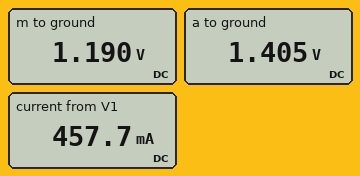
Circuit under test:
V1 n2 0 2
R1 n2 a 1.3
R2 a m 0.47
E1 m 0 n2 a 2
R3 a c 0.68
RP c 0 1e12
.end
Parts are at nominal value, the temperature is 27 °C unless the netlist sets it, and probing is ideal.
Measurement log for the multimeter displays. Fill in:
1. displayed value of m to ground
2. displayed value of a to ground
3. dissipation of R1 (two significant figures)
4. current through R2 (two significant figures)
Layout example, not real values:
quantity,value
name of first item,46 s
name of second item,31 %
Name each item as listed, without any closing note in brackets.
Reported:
quantity,value
displayed value of m to ground,1.190 V
displayed value of a to ground,1.405 V
dissipation of R1,270 mW
current through R2,460 mA
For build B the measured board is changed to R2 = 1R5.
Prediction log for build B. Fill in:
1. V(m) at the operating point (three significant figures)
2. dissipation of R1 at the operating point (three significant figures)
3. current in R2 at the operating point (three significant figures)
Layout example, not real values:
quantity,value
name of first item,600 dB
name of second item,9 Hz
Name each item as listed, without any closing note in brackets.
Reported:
quantity,value
V(m) at the operating point,963 mV
dissipation of R1 at the operating point,178 mW
current in R2 at the operating point,370 mA
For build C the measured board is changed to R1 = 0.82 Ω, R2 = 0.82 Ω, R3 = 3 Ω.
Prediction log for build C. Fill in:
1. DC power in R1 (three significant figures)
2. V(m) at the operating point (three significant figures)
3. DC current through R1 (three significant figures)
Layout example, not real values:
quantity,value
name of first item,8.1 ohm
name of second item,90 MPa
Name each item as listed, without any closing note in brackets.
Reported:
quantity,value
DC power in R1,305 mW
V(m) at the operating point,1.00 V
DC current through R1,610 mA
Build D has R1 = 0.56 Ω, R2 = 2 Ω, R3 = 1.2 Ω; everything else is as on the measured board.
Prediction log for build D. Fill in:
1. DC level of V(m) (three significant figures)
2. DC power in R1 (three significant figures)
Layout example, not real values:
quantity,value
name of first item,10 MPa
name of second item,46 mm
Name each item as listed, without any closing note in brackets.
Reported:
quantity,value
DC level of V(m),609 mV
DC power in R1,165 mW
